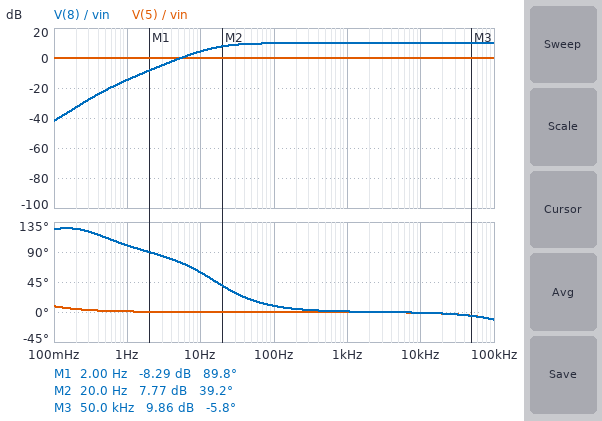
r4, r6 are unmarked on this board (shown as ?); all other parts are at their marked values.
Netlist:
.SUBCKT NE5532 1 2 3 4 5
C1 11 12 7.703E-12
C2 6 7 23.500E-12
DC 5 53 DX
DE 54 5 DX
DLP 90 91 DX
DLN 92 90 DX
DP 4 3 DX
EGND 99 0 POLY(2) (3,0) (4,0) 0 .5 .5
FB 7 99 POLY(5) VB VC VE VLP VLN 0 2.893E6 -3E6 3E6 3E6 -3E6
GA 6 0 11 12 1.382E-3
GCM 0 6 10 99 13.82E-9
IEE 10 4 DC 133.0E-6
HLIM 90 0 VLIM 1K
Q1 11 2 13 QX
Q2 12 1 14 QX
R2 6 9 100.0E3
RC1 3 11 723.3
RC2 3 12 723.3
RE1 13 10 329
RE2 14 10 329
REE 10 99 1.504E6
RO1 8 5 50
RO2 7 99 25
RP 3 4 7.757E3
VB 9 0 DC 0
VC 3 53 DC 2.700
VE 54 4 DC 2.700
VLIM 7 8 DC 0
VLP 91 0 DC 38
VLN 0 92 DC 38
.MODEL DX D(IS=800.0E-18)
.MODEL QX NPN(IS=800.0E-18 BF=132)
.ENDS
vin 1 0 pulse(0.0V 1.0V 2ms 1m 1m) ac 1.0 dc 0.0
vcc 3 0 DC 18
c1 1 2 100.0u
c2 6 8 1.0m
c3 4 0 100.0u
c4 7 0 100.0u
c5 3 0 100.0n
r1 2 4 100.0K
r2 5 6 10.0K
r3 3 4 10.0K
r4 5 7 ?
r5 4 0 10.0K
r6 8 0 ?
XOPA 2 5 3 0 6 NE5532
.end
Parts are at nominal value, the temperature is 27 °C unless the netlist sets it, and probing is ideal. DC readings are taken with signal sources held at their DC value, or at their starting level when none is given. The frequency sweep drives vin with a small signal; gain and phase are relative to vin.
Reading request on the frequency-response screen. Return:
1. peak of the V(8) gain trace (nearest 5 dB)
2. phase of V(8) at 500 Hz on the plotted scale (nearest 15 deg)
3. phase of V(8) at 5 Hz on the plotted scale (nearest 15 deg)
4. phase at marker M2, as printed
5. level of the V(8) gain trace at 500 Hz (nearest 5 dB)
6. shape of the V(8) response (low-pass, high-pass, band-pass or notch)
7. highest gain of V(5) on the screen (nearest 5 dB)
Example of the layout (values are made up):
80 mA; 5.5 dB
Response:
10 dB; 0 deg; 75 deg; 39.2 deg; 10 dB; high-pass; 0 dB
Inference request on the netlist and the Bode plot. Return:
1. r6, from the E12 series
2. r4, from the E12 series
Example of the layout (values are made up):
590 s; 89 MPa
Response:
10 Ω; 4.7 kΩ
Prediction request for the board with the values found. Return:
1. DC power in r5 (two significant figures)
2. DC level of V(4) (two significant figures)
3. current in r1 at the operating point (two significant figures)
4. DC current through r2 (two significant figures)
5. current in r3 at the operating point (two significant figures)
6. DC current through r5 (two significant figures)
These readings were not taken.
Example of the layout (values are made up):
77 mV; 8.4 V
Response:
8.1 mW; 9.0 V; 500 nA; 500 nA; 900 µA; 900 µA
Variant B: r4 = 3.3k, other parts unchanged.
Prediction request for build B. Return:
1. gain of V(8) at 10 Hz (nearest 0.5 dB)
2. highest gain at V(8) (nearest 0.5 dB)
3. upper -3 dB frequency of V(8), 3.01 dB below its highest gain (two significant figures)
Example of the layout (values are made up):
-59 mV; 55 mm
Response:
6.5 dB; 12.0 dB; 390 kHz
